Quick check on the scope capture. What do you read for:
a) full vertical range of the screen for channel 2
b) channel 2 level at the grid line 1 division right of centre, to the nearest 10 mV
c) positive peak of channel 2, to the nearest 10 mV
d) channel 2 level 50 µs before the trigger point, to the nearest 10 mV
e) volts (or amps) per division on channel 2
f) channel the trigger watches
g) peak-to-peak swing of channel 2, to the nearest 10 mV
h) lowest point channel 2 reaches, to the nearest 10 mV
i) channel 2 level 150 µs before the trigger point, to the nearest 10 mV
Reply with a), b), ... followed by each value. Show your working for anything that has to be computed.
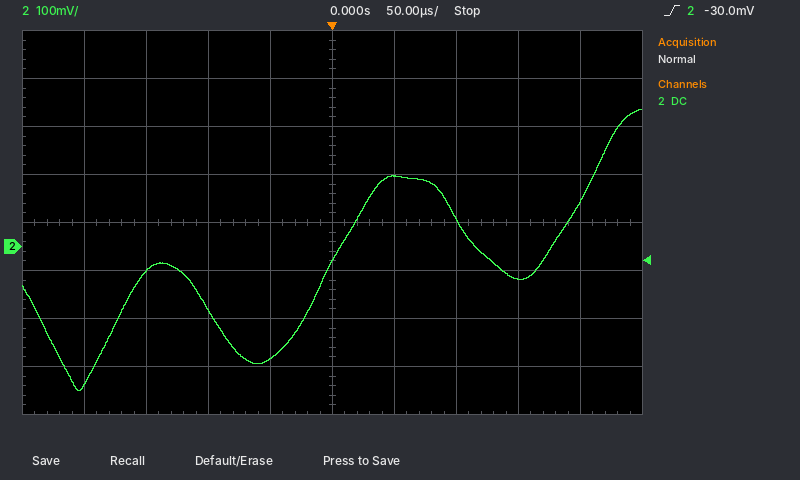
a) 800 mV
b) 150 mV
c) 290 mV
d) -230 mV
e) 100 mV
f) channel 2
g) 290 mV − (-300 mV) = 590 mV
h) -300 mV
i) -50 mV
